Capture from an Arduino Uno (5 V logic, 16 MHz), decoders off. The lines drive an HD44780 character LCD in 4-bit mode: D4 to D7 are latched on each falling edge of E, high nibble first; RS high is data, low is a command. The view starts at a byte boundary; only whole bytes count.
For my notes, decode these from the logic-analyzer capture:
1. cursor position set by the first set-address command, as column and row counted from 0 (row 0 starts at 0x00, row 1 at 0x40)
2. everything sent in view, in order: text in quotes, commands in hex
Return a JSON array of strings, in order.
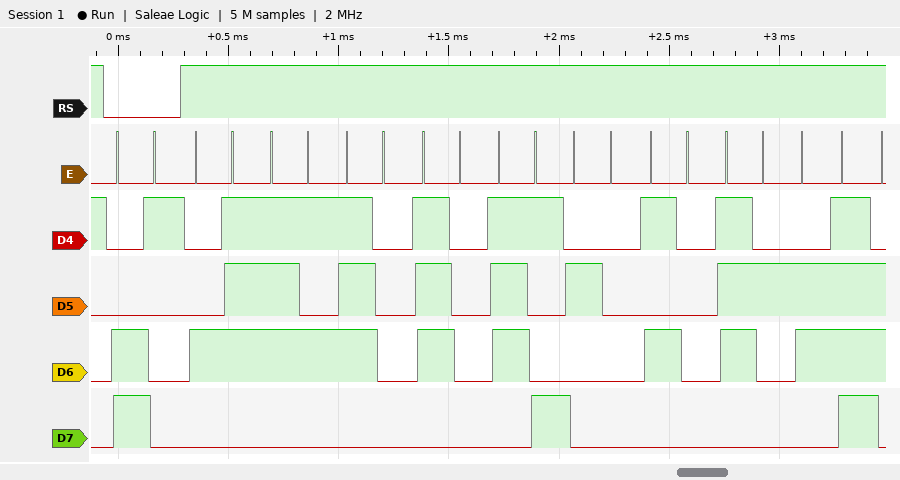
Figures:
["column 1, row 1", "0xC1 \"Guppy Pro\""]
